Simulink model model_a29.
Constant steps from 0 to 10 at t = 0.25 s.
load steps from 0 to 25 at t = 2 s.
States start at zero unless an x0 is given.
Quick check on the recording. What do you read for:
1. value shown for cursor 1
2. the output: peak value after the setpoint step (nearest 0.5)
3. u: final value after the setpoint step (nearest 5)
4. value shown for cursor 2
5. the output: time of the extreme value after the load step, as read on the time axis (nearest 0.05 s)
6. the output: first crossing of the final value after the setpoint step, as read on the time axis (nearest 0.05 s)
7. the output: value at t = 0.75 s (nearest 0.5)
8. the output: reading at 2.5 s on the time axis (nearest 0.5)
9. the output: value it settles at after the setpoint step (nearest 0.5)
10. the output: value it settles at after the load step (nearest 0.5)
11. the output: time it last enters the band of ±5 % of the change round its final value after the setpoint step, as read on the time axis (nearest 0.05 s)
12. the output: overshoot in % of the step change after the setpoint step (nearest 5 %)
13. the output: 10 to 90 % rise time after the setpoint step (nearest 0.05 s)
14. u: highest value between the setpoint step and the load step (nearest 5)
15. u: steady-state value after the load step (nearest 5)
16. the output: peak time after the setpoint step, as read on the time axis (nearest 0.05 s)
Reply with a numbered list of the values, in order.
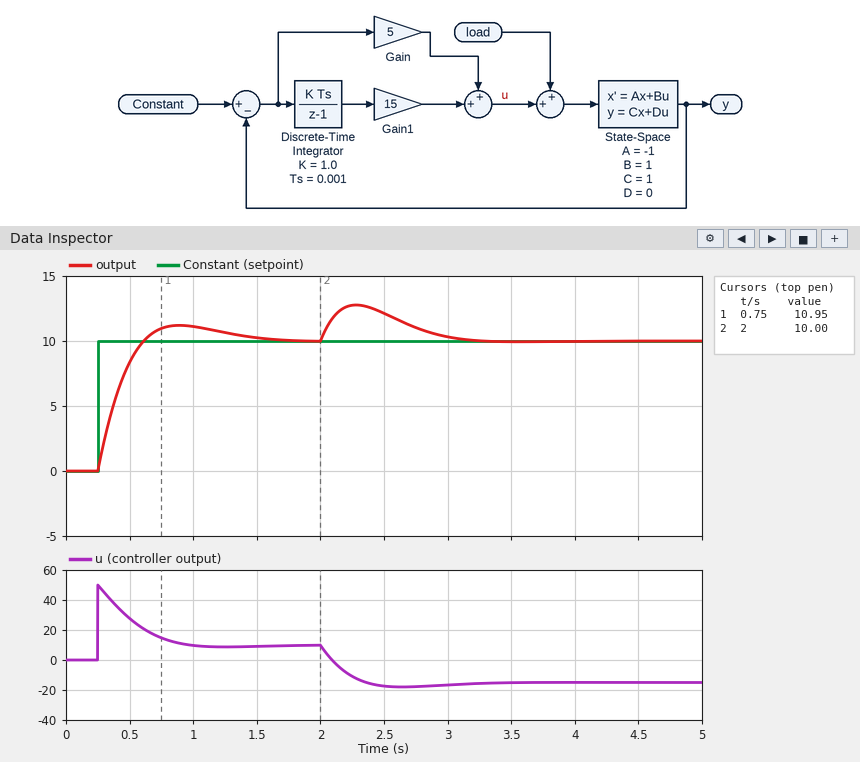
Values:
1. 10.95
2. 11.0
3. 10
4. 10.00
5. 2.30 s
6. 0.60 s
7. 11.0
8. 12.0
9. 10.0
10. 10.0
11. 1.35 s
12. 10 %
13. 0.25 s
14. 50
15. -15
16. 0.90 s
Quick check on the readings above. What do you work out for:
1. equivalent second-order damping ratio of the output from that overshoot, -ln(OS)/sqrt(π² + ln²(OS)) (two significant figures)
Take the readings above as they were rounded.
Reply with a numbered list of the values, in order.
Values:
1. 0.59
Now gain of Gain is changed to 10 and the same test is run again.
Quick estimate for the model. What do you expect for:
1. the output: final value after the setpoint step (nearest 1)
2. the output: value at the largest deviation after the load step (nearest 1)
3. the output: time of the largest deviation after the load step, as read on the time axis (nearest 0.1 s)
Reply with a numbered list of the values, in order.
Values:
1. 10
2. 12
3. 2.2 s
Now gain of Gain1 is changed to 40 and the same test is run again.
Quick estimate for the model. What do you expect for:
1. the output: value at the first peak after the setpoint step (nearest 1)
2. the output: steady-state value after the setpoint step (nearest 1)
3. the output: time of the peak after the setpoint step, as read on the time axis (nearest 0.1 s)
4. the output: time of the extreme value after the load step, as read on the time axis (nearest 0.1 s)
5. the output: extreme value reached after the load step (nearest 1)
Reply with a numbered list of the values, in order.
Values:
1. 13
2. 10
3. 0.7 s
4. 2.2 s
5. 12
